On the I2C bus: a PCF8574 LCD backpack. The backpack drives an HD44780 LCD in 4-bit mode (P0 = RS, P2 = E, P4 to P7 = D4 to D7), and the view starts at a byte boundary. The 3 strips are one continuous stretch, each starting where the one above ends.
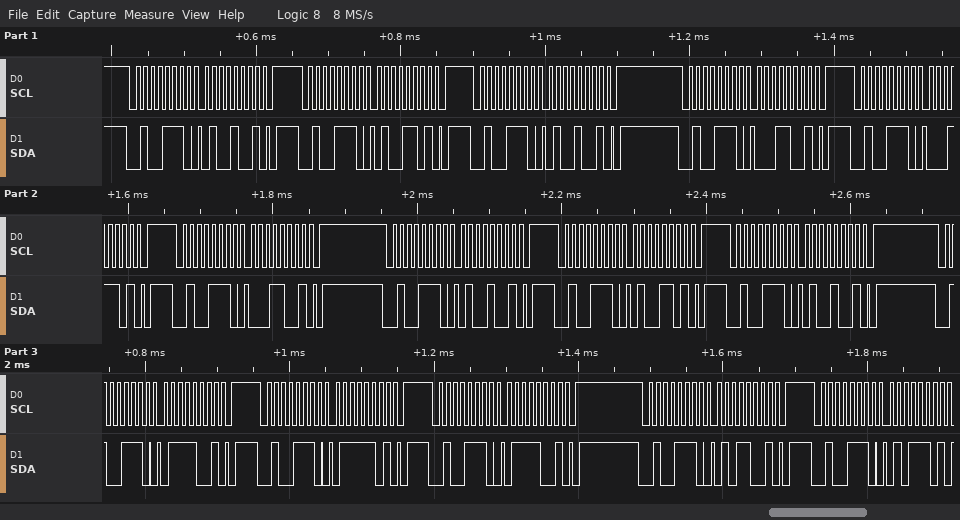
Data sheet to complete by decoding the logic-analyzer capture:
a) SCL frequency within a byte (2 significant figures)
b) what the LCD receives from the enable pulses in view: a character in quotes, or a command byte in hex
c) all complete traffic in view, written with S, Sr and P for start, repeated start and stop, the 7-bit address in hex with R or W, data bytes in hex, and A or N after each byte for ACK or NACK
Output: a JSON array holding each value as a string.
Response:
["100 kHz", "'A' 'G'", "S 27W A 49 A P S 27W A 4D A P S 27W A 49 A P S 27W A 19 A P S 27W A 1D A P S 27W A 19 A P S 27W A 49 A P S 27W A 4D A P S 27W A 49 A P S 27W A 79 A P S 27W A 7D A P S 27W A 79 A P S 27W A 59 A P S 27W A 5D A"]
